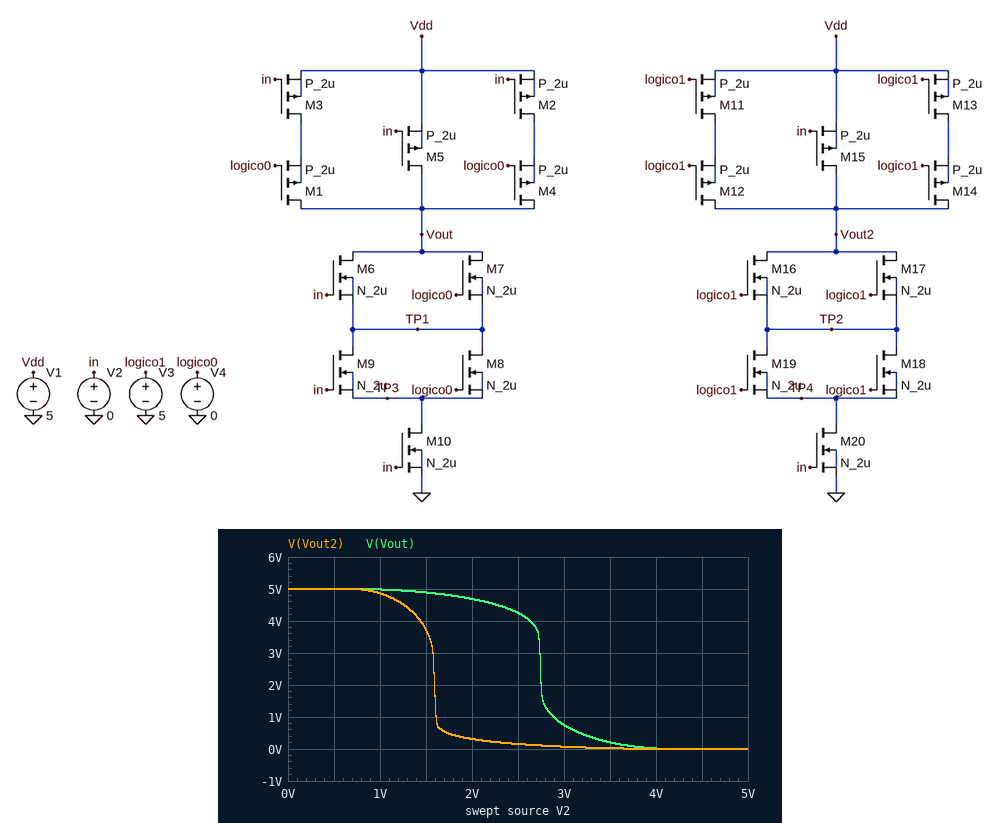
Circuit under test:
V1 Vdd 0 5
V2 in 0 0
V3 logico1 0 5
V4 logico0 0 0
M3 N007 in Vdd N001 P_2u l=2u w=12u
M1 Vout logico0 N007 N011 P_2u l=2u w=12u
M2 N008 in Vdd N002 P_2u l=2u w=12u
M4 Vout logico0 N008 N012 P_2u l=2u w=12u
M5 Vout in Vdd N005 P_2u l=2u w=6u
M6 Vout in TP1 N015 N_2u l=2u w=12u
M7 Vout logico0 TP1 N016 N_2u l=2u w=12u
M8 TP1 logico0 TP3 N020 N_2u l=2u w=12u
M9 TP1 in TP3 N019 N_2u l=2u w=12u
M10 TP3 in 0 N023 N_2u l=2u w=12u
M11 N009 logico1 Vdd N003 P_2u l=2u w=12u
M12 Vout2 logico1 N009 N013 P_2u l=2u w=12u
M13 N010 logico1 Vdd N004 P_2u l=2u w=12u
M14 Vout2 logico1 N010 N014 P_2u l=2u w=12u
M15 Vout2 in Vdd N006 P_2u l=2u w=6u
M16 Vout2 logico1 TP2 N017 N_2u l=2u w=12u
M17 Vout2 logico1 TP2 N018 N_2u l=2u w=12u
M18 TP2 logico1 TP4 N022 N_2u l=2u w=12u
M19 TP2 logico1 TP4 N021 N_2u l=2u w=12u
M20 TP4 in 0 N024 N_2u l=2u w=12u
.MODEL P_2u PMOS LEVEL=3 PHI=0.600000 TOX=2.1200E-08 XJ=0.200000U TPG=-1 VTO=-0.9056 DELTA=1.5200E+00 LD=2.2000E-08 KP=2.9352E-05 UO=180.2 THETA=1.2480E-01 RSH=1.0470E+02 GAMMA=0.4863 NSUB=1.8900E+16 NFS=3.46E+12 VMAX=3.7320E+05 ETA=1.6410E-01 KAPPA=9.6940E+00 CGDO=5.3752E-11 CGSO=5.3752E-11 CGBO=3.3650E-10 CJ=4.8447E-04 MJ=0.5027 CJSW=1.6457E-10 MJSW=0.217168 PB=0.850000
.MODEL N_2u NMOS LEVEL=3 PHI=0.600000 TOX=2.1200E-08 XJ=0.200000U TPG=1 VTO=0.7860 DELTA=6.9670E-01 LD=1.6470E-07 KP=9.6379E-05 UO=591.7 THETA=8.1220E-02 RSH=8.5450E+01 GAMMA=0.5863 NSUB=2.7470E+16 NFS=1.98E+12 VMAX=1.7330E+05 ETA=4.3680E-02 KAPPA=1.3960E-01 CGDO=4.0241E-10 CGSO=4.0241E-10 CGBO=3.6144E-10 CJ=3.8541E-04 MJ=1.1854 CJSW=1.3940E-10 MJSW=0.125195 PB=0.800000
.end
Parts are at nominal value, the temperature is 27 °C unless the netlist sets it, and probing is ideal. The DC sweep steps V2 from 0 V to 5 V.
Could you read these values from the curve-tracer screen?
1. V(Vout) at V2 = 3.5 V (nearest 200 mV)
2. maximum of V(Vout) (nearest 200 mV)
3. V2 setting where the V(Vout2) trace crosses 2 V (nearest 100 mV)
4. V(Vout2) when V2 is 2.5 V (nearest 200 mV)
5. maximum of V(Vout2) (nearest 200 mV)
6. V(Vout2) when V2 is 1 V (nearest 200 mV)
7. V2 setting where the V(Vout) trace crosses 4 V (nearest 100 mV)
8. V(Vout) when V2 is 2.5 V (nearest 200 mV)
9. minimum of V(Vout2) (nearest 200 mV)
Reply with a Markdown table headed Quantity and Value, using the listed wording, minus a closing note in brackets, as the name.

| Quantity | Value |
|---|---|
| V(Vout) at V2 = 3.5 V | 200 mV |
| maximum of V(Vout) | 5.0 V |
| V2 setting where the V(Vout2) trace crosses 2 V | 1.6 V |
| V(Vout2) when V2 is 2.5 V | 200 mV |
| maximum of V(Vout2) | 5.0 V |
| V(Vout2) when V2 is 1 V | 4.8 V |
| V2 setting where the V(Vout) trace crosses 4 V | 2.6 V |
| V(Vout) when V2 is 2.5 V | 4.2 V |
| minimum of V(Vout2) | 0 V |
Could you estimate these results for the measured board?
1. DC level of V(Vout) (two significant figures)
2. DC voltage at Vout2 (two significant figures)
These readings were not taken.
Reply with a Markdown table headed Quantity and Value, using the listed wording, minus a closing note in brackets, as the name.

| Quantity | Value |
|---|---|
| DC level of V(Vout) | 5.0 V |
| DC voltage at Vout2 | 5.0 V |
